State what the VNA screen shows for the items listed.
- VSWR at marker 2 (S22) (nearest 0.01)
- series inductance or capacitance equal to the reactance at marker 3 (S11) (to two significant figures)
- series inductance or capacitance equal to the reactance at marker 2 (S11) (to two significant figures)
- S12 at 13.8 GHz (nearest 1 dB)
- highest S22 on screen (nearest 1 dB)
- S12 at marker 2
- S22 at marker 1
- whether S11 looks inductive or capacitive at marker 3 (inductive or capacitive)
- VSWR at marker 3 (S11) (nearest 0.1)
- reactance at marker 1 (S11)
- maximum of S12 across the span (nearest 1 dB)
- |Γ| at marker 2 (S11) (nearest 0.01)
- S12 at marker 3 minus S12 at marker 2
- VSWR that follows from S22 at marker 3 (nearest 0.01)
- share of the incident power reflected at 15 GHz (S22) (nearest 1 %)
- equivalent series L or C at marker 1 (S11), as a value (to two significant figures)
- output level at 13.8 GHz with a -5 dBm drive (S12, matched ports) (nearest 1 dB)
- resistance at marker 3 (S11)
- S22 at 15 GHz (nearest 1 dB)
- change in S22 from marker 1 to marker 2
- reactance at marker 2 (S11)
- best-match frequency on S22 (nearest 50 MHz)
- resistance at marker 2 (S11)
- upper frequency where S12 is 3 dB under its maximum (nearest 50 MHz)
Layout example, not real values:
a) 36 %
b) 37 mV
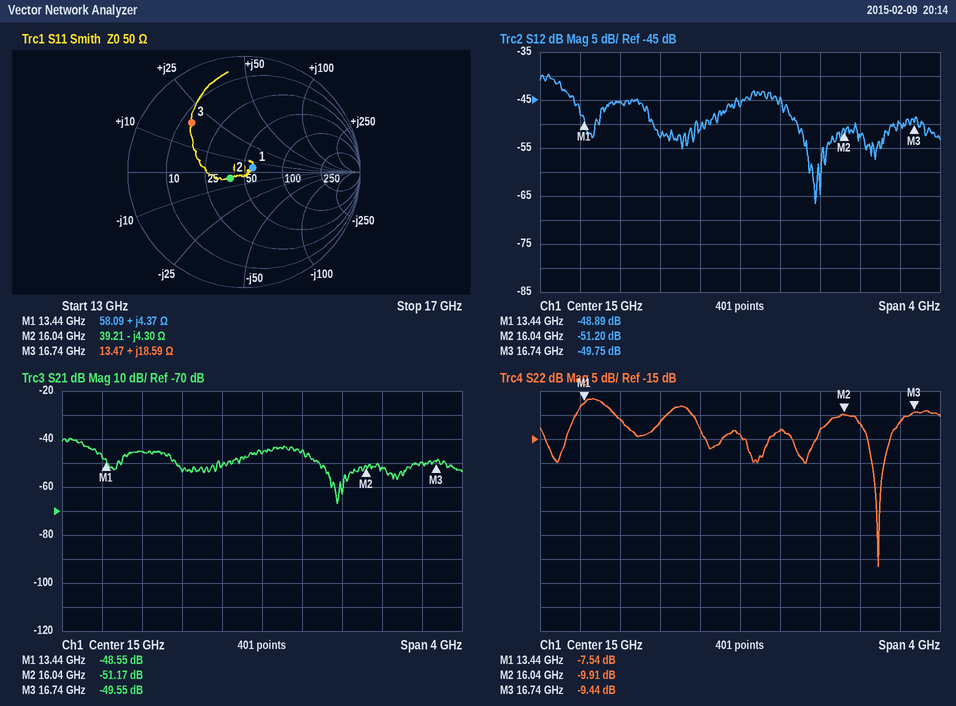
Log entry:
a) 1.94
b) 180 pH
c) 2.3 pF
d) -45 dB
e) -7 dB
f) -51.20 dB
g) -7.54 dB
h) inductive
i) 4.3
j) +4.37 Ω
k) -40 dB
l) 0.13
m) 1.45 dB
n) 2.02
o) 4 %
p) 52 pH
q) -50 dBm
r) 13.47 Ω
s) -14 dB
t) -2.37 dB
u) -4.30 Ω
v) 16.40 GHz
w) 39.21 Ω
x) 13.20 GHz
